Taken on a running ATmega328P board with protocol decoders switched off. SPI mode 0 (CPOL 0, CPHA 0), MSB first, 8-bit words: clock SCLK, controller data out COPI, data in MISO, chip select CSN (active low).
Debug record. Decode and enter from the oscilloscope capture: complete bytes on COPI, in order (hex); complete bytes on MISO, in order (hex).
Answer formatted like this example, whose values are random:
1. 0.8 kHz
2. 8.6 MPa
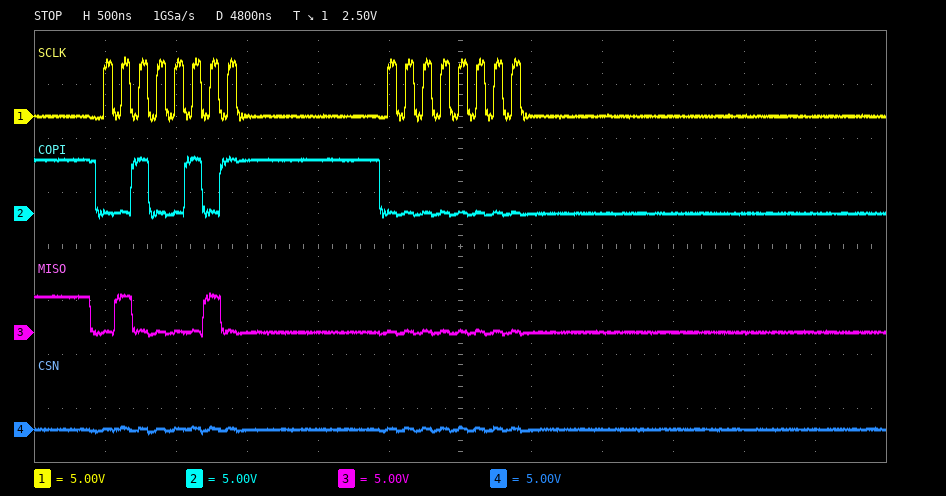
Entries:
1. 25 00
2. 42 00
